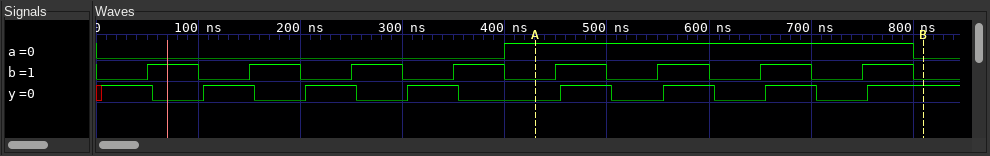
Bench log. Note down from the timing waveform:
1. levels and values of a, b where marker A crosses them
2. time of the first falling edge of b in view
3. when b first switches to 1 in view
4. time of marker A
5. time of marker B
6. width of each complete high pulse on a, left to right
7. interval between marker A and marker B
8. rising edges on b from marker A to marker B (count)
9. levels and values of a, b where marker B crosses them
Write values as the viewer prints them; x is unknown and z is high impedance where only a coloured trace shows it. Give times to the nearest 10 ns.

a=1, b=0
100 ns
50 ns
430 ns
810 ns
400 ns
380 ns
4
a=0, b=0
